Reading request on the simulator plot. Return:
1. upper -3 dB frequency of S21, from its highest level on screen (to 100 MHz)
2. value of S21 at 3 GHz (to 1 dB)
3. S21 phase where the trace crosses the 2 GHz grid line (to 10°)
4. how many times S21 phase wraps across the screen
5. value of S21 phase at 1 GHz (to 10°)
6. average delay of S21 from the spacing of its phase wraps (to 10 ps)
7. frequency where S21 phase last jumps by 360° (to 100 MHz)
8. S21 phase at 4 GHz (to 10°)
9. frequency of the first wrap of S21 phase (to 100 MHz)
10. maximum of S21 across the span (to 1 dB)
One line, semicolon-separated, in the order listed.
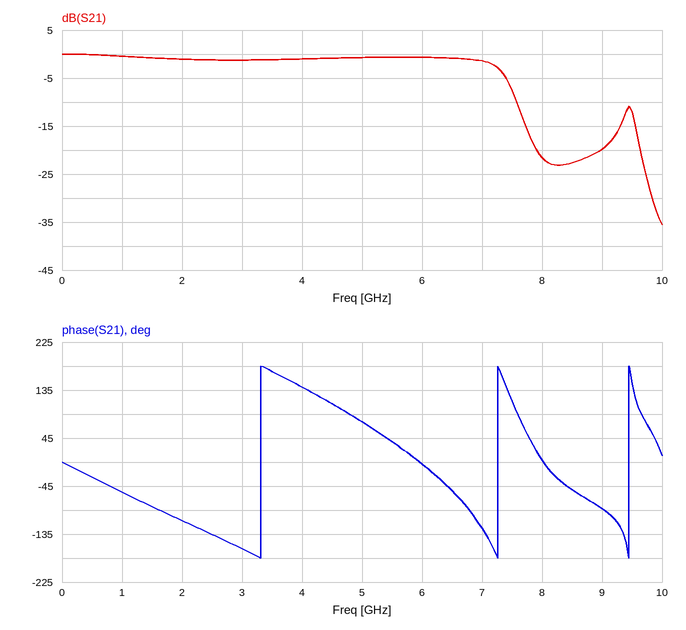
7.3 GHz; -1 dB; -110°; 3; -60°; 330 ps; 9.4 GHz; 140°; 3.3 GHz; 0 dB
